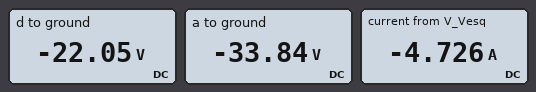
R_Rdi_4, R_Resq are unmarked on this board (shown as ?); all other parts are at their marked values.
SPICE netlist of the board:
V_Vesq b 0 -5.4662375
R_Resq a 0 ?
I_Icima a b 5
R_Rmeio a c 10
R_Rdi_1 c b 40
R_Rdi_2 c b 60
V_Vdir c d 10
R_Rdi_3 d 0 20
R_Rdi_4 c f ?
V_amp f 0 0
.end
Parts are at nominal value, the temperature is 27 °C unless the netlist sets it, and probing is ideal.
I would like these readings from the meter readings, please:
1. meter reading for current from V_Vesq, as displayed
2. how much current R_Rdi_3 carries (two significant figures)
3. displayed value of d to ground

-4.726 A
1.1 A
-22.05 V
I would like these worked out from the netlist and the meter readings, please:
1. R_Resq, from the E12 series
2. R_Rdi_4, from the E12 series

12 Ω
15 Ω
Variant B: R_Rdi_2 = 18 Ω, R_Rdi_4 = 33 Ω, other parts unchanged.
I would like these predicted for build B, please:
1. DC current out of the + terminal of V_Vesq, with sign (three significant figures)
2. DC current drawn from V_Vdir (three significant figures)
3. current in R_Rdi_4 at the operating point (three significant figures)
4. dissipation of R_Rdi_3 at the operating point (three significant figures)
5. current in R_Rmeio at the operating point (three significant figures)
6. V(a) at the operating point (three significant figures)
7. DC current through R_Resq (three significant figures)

-4.40 A
1.15 A
392 mA
26.3 W
2.14 A
-34.3 V
2.86 A
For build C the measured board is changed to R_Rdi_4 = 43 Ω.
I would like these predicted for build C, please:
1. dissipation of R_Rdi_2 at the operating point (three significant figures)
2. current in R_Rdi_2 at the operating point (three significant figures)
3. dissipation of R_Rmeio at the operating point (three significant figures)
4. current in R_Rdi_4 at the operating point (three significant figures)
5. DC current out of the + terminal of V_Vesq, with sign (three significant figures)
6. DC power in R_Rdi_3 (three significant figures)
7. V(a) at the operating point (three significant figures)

1.61 W
164 mA
41.3 W
356 mA
-4.59 A
32.0 W
-35.6 V
